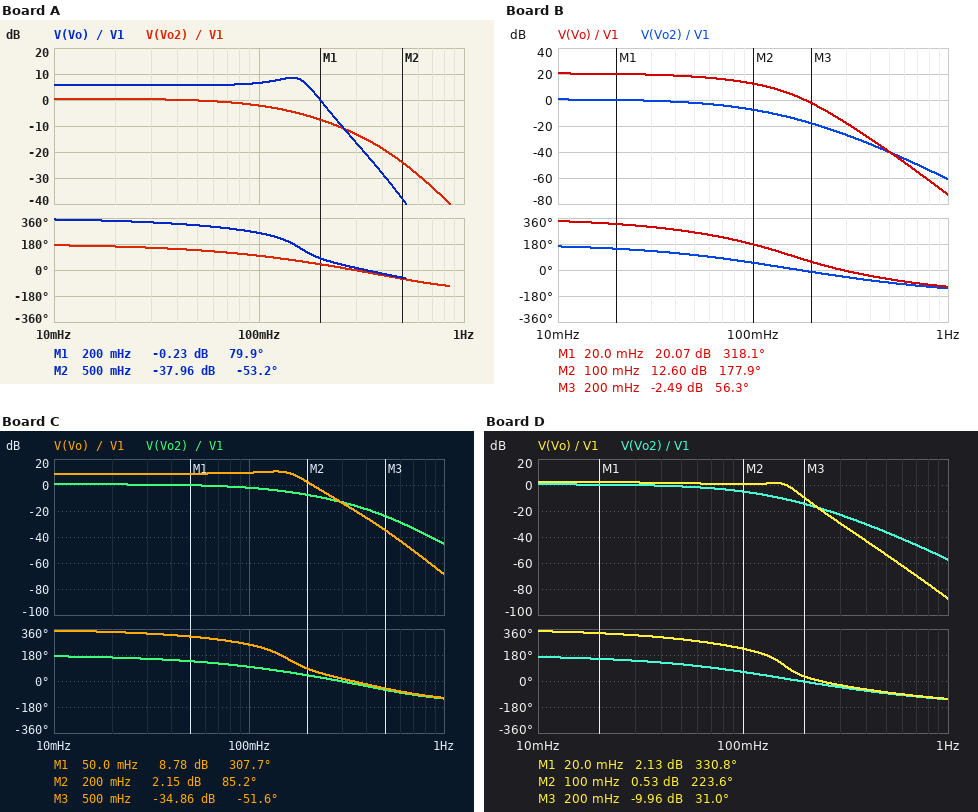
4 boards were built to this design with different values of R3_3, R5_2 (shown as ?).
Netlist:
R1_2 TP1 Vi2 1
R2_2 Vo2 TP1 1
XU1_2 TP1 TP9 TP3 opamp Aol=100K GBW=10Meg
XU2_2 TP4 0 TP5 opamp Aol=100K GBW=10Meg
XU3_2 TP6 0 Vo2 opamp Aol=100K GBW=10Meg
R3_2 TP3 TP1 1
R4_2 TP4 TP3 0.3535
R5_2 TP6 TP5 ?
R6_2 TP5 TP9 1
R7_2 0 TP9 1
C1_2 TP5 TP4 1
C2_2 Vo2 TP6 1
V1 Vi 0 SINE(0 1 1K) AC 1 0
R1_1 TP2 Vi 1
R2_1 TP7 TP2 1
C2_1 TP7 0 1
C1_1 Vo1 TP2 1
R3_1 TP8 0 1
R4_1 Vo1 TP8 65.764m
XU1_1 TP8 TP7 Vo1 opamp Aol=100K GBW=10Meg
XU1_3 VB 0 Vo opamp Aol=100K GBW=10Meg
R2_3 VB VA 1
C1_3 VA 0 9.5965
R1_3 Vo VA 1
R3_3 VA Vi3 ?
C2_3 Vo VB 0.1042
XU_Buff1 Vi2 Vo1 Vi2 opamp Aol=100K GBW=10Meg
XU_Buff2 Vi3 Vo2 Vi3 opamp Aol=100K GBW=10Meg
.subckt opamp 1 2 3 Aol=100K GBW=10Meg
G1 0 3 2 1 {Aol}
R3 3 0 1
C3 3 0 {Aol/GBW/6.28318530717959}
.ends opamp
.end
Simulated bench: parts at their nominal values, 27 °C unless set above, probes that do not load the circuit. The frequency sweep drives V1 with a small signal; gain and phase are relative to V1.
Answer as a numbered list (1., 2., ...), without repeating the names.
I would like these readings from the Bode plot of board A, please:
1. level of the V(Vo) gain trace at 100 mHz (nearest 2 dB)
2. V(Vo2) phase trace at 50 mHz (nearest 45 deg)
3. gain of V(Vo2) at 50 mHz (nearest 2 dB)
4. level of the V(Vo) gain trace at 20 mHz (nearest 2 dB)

1. 6 dB
2. 135 deg
3. 0 dB
4. 6 dB
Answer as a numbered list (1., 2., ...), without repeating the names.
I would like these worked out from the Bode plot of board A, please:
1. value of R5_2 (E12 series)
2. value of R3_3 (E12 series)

1. 0.33 Ω
2. 0.56 Ω
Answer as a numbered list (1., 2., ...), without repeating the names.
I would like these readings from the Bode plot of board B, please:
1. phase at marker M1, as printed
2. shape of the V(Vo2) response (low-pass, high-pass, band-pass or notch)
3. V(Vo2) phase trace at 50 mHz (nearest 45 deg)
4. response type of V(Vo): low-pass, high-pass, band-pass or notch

1. 318.1 deg
2. low-pass
3. 90 deg
4. low-pass
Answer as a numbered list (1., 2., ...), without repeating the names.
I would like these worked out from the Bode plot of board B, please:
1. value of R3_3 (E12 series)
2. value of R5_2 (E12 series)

1. 0.1 Ω
2. 1.8 Ω
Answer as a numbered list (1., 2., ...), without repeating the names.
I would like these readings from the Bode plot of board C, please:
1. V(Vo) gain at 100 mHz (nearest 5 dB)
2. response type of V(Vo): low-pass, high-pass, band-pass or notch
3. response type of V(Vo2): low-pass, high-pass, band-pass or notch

1. 10 dB
2. low-pass
3. low-pass
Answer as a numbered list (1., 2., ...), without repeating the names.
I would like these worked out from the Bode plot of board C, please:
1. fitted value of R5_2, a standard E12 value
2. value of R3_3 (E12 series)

1. 0.33 Ω
2. 0.39 Ω
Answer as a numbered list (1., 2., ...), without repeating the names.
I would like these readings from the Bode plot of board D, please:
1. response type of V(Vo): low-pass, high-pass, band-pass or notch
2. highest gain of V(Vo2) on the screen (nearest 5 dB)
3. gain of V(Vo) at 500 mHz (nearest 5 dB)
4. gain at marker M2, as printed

1. low-pass
2. 0 dB
3. -55 dB
4. 0.53 dB
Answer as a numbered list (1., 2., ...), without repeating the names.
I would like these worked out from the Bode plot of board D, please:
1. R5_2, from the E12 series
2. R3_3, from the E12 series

1. 1.2 Ω
2. 0.82 Ω
